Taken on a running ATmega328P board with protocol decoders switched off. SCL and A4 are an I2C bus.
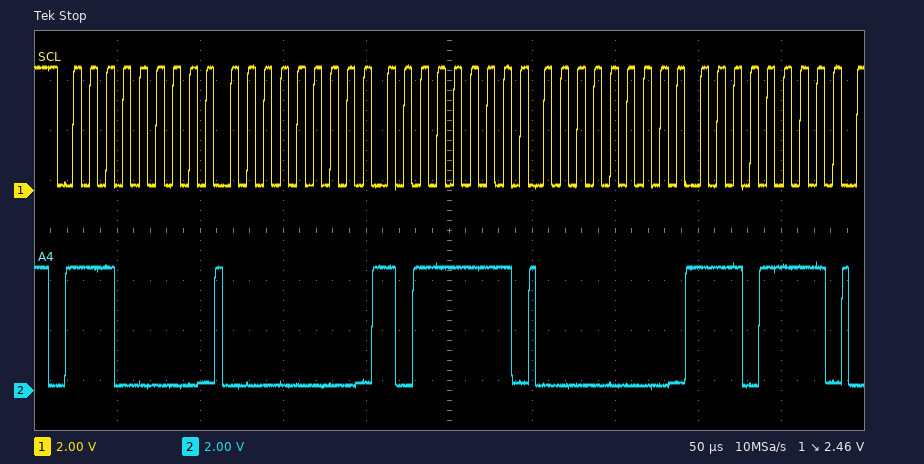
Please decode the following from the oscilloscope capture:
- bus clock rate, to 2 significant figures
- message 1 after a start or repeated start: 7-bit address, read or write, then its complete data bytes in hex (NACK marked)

100 kHz
0x70 write: 00 BF 00 EF
